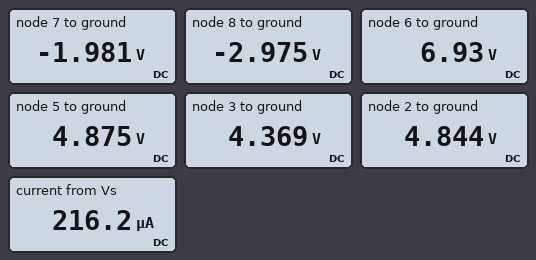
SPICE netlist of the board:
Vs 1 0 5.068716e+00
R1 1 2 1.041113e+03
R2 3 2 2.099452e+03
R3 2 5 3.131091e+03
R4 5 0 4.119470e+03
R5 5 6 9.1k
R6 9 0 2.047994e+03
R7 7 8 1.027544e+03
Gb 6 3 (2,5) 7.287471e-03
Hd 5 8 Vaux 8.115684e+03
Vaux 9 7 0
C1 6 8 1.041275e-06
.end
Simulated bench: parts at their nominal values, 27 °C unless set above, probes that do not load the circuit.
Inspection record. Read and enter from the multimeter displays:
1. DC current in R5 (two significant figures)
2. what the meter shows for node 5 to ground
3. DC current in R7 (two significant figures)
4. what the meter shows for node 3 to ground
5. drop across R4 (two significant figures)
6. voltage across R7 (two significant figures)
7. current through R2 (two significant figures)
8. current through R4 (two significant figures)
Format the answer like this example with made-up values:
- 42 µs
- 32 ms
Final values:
- 230 µA
- 4.875 V
- 970 µA
- 4.369 V
- 4.9 V
- 990 mV
- 230 µA
- 1.2 mA
